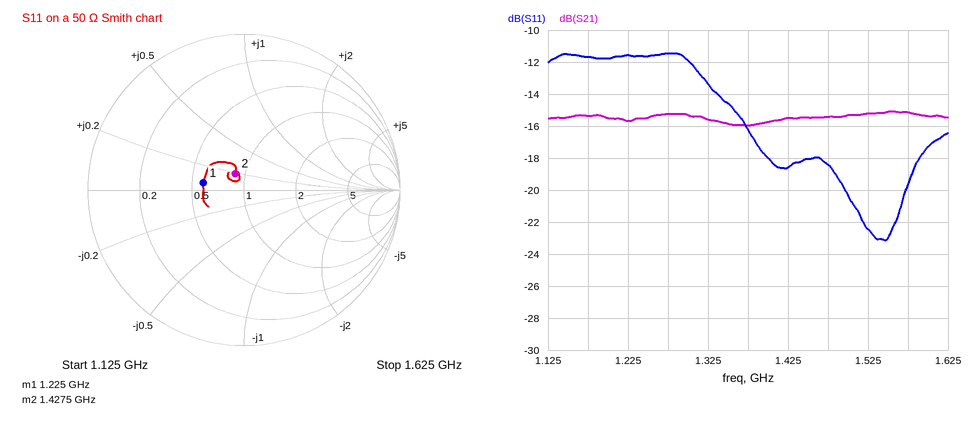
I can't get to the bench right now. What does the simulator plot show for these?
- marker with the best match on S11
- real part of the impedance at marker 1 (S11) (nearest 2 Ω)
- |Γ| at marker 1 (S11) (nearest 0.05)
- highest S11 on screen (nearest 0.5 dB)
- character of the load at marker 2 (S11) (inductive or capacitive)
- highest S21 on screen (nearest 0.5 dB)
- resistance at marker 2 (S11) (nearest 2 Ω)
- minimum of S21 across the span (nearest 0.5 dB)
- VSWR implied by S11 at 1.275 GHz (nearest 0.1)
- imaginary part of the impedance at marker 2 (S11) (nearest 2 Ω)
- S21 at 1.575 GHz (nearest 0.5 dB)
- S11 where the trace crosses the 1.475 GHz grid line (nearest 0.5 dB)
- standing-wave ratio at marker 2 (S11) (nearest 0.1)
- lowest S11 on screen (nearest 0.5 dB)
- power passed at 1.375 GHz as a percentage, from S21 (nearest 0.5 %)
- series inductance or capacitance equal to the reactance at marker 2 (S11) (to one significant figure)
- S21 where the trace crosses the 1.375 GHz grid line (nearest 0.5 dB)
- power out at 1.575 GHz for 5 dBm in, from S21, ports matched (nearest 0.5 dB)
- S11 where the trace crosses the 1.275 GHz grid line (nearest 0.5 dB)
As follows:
marker 2
30 Ω
0.25
-11.5 dB
inductive
-15.0 dB
44 Ω
-16.0 dB
1.7
+10 Ω
-15.0 dB
-18.5 dB
1.3
-23.0 dB
2.5 %
1 nH
-16.0 dB
-10.0 dBm
-11.5 dB
